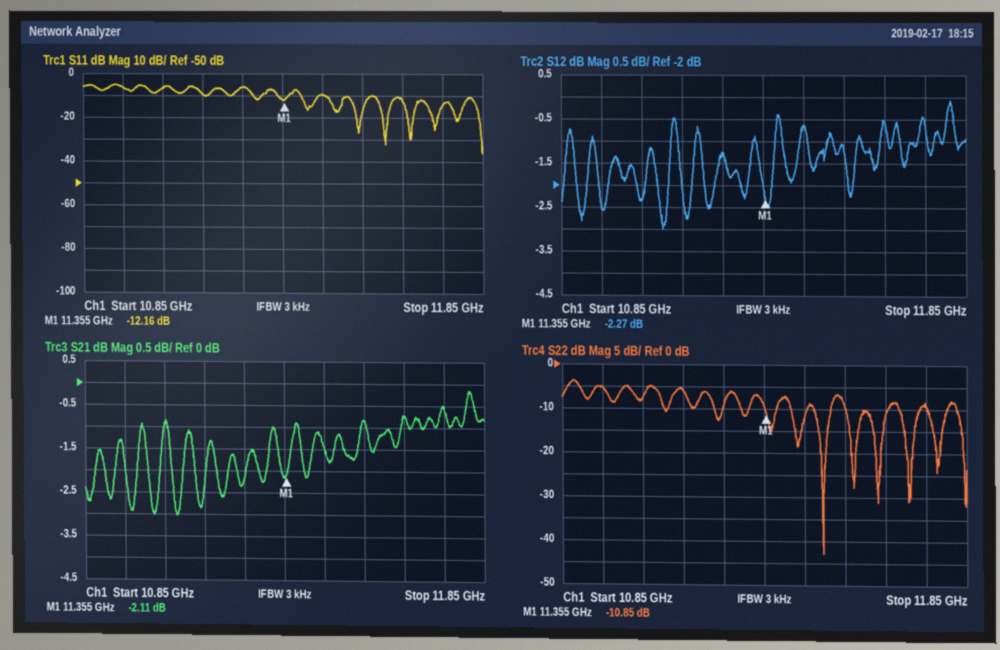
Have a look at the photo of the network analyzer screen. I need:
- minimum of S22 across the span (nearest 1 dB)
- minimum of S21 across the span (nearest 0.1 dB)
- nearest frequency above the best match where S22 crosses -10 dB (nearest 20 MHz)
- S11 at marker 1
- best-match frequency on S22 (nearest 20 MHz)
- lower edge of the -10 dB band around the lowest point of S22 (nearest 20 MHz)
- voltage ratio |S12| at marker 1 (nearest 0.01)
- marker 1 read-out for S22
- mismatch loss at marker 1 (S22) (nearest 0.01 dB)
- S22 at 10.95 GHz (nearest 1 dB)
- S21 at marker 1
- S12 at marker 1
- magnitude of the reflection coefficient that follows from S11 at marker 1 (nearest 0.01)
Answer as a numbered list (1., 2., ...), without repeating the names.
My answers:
1. -43 dB
2. -3.0 dB
3. 11.52 GHz
4. -12.16 dB
5. 11.50 GHz
6. 11.48 GHz
7. 0.77
8. -10.85 dB
9. 0.37 dB
10. -5 dB
11. -2.11 dB
12. -2.27 dB
13. 0.25
